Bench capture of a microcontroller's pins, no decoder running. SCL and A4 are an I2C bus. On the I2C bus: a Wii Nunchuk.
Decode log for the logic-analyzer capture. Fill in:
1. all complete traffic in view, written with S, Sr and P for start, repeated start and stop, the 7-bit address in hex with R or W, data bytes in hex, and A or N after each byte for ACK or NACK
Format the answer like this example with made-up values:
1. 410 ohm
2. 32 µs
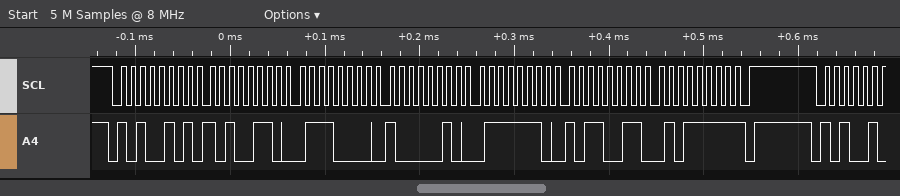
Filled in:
1. S 52R A A6 A 70 A 82 A 7E A B3 A 5F N P
